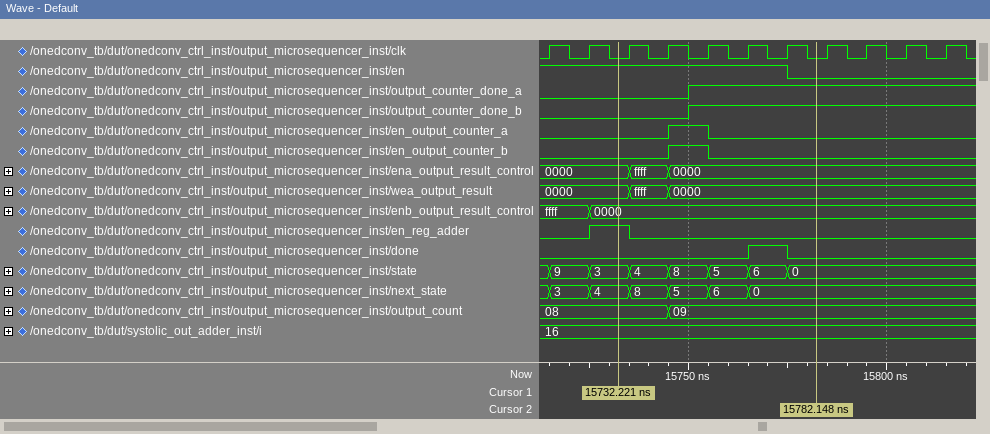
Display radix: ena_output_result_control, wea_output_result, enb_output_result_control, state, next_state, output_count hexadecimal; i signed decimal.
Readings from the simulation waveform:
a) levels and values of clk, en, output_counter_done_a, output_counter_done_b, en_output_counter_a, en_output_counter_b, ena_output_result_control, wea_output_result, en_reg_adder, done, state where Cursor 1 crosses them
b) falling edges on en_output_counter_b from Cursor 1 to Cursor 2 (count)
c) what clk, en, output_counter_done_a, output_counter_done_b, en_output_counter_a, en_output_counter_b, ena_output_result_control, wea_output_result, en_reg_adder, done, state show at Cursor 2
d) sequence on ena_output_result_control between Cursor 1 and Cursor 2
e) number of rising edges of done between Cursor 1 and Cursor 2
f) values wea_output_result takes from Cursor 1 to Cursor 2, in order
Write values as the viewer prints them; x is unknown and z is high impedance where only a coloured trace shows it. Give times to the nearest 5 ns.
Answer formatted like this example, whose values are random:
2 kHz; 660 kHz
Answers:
clk=0, en=1, output_counter_done_a=0, output_counter_done_b=0, en_output_counter_a=0, en_output_counter_b=0, ena_output_result_control=0000, wea_output_result=0000, en_reg_adder=1, done=0, state=3; 1; clk=0, en=0, output_counter_done_a=1, output_counter_done_b=1, en_output_counter_a=0, en_output_counter_b=0, ena_output_result_control=0000, wea_output_result=0000, en_reg_adder=0, done=0, state=0; 0000, ffff, 0000; 1; 0000, ffff, 0000
